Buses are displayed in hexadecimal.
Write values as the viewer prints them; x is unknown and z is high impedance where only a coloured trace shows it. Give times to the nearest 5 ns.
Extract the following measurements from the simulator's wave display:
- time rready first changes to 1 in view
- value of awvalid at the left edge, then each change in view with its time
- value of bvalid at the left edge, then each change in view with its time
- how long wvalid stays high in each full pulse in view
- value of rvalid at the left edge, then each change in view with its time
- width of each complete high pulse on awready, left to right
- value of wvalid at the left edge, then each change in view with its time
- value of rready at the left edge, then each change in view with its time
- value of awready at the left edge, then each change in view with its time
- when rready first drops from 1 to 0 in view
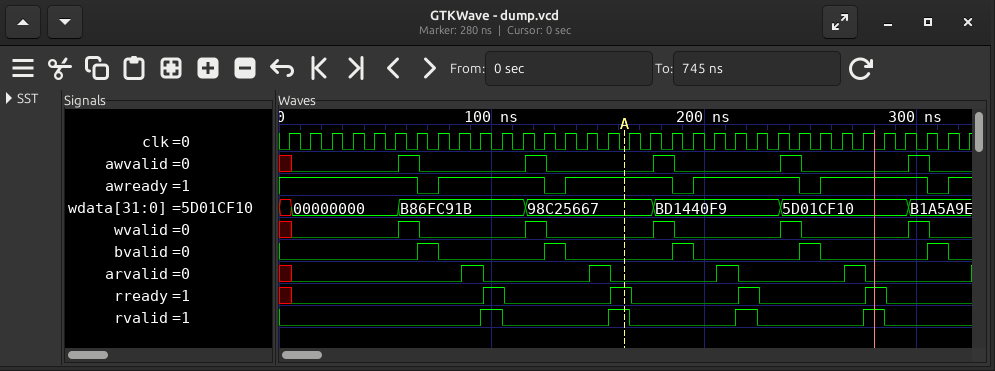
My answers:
95 ns
x, 0 at 5 ns, 1 at 55 ns, 0 at 65 ns, 1 at 115 ns, 0 at 125 ns, 1 at 175 ns, 0 at 185 ns, 1 at 235 ns, 0 at 245 ns, 1 at 295 ns, 0 at 305 ns
0, 1 at 65 ns, 0 at 75 ns, 1 at 125 ns, 0 at 135 ns, 1 at 185 ns, 0 at 195 ns, 1 at 245 ns, 0 at 255 ns, 1 at 305 ns, 0 at 315 ns
10 ns, 10 ns, 10 ns, 10 ns, 10 ns
0, 1 at 95 ns, 0 at 105 ns, 1 at 155 ns, 0 at 165 ns, 1 at 215 ns, 0 at 225 ns, 1 at 275 ns, 0 at 285 ns
50 ns, 50 ns, 50 ns, 50 ns
x, 0 at 5 ns, 1 at 55 ns, 0 at 65 ns, 1 at 115 ns, 0 at 125 ns, 1 at 175 ns, 0 at 185 ns, 1 at 235 ns, 0 at 245 ns, 1 at 295 ns, 0 at 305 ns
x, 0 at 5 ns, 1 at 95 ns, 0 at 105 ns, 1 at 155 ns, 0 at 165 ns, 1 at 215 ns, 0 at 225 ns, 1 at 275 ns, 0 at 285 ns
1, 0 at 65 ns, 1 at 75 ns, 0 at 125 ns, 1 at 135 ns, 0 at 185 ns, 1 at 195 ns, 0 at 245 ns, 1 at 255 ns, 0 at 305 ns, 1 at 315 ns
105 ns
